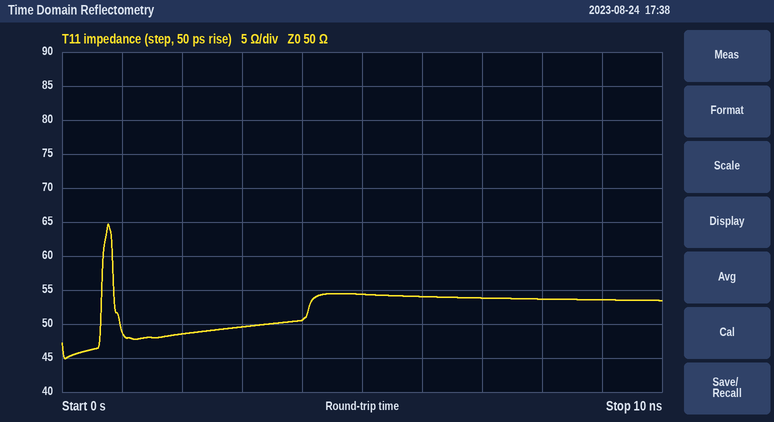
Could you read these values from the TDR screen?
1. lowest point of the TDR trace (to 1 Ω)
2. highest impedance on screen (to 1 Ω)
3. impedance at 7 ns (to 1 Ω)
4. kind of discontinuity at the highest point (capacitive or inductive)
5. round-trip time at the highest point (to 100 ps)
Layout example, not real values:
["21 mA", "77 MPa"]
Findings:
["45 Ω", "65 Ω", "54 Ω", "inductive", "800 ps"]
